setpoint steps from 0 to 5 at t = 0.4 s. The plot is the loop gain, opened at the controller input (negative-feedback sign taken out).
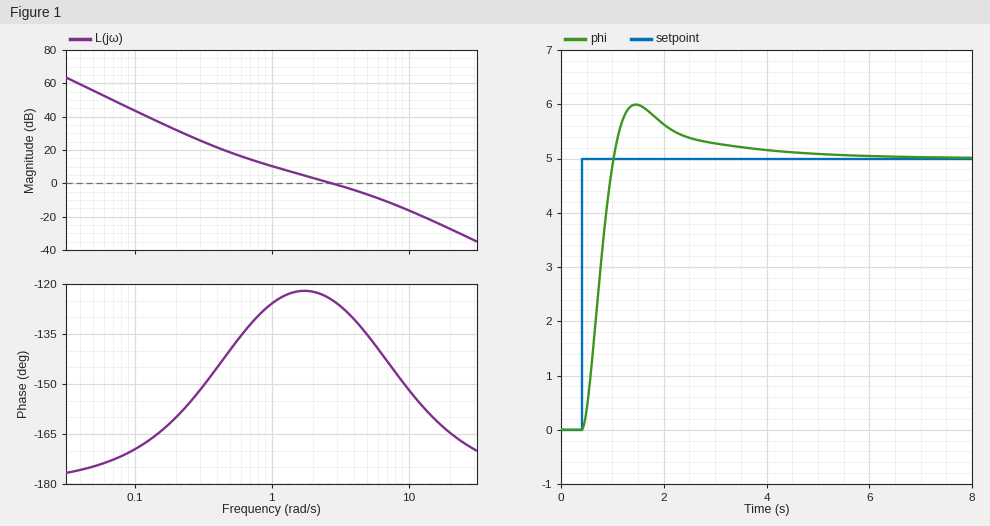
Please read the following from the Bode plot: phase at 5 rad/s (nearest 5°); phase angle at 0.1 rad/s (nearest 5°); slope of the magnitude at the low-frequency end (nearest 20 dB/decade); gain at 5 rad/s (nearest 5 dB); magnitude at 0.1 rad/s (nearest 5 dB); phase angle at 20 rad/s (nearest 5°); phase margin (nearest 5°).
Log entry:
-135°
-170°
-40 dB/decade
-5 dB
45 dB
-165°
55°
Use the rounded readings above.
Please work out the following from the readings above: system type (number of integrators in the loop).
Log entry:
2
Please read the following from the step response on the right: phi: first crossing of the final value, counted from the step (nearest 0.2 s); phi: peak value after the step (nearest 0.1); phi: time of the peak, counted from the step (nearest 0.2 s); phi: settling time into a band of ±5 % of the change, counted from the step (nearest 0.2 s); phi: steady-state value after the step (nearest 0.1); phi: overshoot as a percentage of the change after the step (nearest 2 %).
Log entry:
0.6 s
6.0
1.0 s
2.8 s
5.0
20 %
